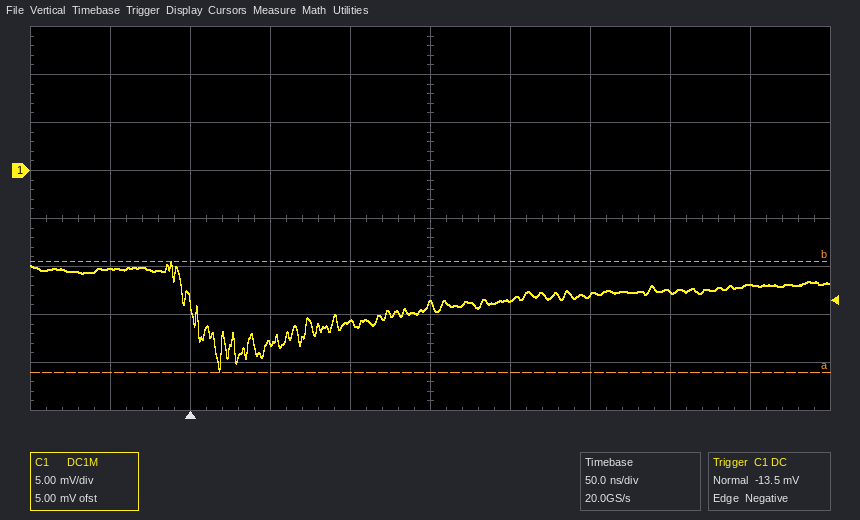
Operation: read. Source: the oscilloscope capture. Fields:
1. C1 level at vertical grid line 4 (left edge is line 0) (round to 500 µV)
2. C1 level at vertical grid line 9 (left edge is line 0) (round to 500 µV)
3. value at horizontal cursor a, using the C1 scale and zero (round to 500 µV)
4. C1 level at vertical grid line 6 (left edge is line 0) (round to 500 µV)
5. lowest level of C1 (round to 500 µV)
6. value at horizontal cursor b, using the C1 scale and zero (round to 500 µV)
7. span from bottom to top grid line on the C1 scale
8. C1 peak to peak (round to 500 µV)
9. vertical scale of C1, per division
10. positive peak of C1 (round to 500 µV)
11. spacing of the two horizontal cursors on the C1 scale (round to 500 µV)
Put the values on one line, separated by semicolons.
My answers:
-16.0 mV; -12.0 mV; -21.0 mV; -13.5 mV; -21.0 mV; -9.5 mV; 40 mV; 11.5 mV; 5 mV; -9.5 mV; 11.5 mV
